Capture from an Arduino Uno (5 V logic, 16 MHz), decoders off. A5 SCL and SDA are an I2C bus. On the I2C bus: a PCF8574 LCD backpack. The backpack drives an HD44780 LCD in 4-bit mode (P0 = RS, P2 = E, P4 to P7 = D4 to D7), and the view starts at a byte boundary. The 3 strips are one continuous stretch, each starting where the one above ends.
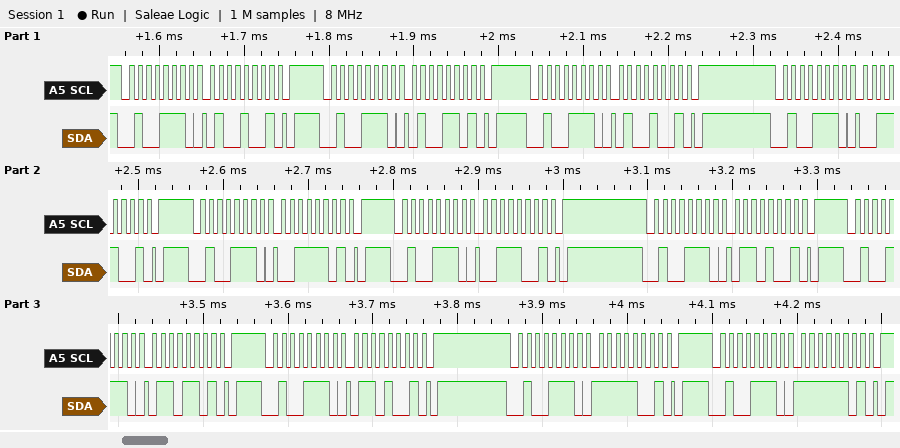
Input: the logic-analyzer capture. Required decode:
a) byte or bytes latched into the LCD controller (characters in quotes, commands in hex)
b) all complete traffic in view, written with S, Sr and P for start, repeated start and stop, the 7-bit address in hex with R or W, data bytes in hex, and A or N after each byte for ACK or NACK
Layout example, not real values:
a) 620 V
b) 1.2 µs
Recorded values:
a) 'C'
b) S 27W A 49 A P S 27W A 4D A P S 27W A 49 A P S 27W A 39 A P S 27W A 3D A P S 27W A 39 A P S 27W A 69 A P S 27W A 6D A P S 27W A 69 A P S 27W A F9 A P S 27W A FD A P
